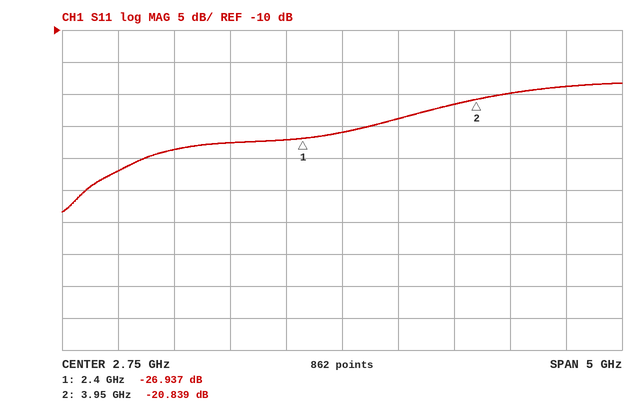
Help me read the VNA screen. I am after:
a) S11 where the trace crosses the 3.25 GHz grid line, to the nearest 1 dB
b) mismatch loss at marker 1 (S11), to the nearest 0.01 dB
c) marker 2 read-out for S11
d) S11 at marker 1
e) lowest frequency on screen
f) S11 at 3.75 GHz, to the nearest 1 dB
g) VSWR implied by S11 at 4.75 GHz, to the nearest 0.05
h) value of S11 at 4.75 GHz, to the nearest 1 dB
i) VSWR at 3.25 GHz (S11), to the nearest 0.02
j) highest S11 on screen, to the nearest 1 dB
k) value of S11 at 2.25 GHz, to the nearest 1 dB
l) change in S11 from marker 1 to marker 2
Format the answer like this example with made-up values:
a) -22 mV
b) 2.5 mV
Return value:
a) -24 dB
b) 0.01 dB
c) -20.839 dB
d) -26.937 dB
e) 250 MHz
f) -22 dB
g) 1.25
h) -19 dB
i) 1.14
j) -18 dB
k) -27 dB
l) 6.098 dB
